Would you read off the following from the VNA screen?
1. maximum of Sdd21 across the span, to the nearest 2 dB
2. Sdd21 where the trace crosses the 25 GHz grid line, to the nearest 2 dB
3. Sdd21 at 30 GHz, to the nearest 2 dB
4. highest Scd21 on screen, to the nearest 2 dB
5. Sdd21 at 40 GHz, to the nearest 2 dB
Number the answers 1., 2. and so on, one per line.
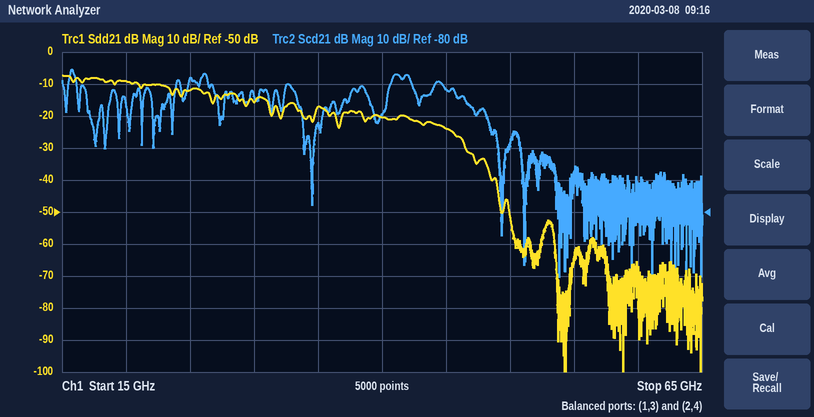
1. -8 dB
2. -12 dB
3. -16 dB
4. -36 dB
5. -20 dB
